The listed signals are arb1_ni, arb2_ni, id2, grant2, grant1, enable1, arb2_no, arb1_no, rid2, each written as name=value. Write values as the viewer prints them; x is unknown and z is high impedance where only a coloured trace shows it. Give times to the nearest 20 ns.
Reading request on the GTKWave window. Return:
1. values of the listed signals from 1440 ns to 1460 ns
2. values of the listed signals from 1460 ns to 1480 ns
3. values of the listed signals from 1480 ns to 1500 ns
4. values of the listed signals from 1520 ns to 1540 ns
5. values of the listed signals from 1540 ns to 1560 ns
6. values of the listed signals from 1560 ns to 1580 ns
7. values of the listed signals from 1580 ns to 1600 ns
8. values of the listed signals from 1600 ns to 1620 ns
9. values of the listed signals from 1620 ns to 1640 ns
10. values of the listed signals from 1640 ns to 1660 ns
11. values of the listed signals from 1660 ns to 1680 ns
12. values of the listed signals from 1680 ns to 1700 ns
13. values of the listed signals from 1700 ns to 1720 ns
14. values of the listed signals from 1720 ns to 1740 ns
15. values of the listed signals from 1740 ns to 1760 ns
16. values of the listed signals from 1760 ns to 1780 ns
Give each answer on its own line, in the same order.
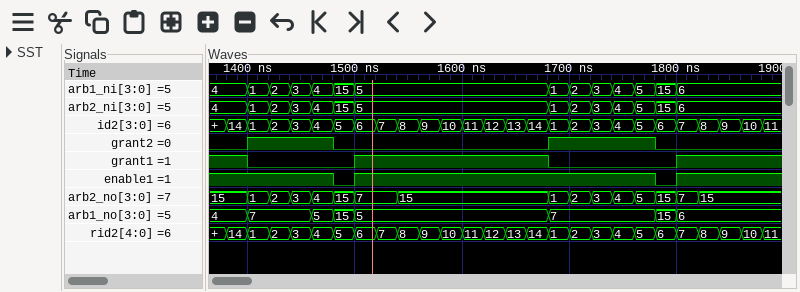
arb1_ni=3, arb2_ni=3, id2=3, grant2=1, grant1=0, enable1=1, arb2_no=3, arb1_no=7, rid2=3
arb1_ni=4, arb2_ni=4, id2=4, grant2=1, grant1=0, enable1=1, arb2_no=4, arb1_no=5, rid2=4
arb1_ni=15, arb2_ni=15, id2=5, grant2=0, grant1=0, enable1=0, arb2_no=15, arb1_no=15, rid2=5
arb1_ni=5, arb2_ni=5, id2=7, grant2=0, grant1=1, enable1=1, arb2_no=7, arb1_no=5, rid2=7
arb1_ni=5, arb2_ni=5, id2=8, grant2=0, grant1=1, enable1=1, arb2_no=15, arb1_no=5, rid2=8
arb1_ni=5, arb2_ni=5, id2=9, grant2=0, grant1=1, enable1=1, arb2_no=15, arb1_no=5, rid2=9
arb1_ni=5, arb2_ni=5, id2=10, grant2=0, grant1=1, enable1=1, arb2_no=15, arb1_no=5, rid2=10
arb1_ni=5, arb2_ni=5, id2=11, grant2=0, grant1=1, enable1=1, arb2_no=15, arb1_no=5, rid2=11
arb1_ni=5, arb2_ni=5, id2=12, grant2=0, grant1=1, enable1=1, arb2_no=15, arb1_no=5, rid2=12
arb1_ni=5, arb2_ni=5, id2=13, grant2=0, grant1=1, enable1=1, arb2_no=15, arb1_no=5, rid2=13
arb1_ni=5, arb2_ni=5, id2=14, grant2=0, grant1=1, enable1=1, arb2_no=15, arb1_no=5, rid2=14
arb1_ni=1, arb2_ni=1, id2=1, grant2=1, grant1=0, enable1=1, arb2_no=1, arb1_no=7, rid2=1
arb1_ni=2, arb2_ni=2, id2=2, grant2=1, grant1=0, enable1=1, arb2_no=2, arb1_no=7, rid2=2
arb1_ni=3, arb2_ni=3, id2=3, grant2=1, grant1=0, enable1=1, arb2_no=3, arb1_no=7, rid2=3
arb1_ni=4, arb2_ni=4, id2=4, grant2=1, grant1=0, enable1=1, arb2_no=4, arb1_no=7, rid2=4
arb1_ni=5, arb2_ni=5, id2=5, grant2=1, grant1=0, enable1=1, arb2_no=5, arb1_no=7, rid2=5
